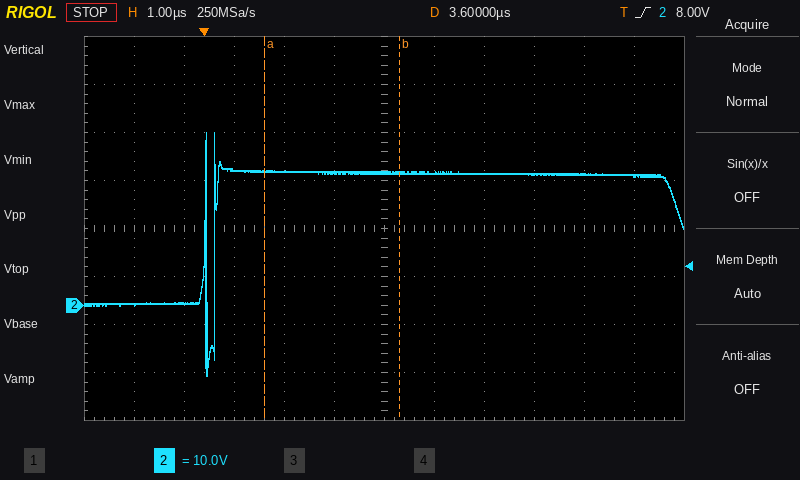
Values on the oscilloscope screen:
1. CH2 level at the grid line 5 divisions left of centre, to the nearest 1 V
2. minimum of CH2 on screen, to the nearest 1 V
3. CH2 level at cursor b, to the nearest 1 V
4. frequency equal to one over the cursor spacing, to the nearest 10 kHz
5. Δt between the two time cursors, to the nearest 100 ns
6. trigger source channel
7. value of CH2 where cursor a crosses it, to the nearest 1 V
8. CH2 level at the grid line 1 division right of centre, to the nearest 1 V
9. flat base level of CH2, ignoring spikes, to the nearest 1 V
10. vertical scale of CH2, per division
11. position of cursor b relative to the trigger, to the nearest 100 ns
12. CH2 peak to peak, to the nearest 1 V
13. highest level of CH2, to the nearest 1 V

0 V
-15 V
28 V
370 kHz
2.7 µs
CH2
28 V
28 V
0 V
10 V
+3.9 µs
51 V
36 V
